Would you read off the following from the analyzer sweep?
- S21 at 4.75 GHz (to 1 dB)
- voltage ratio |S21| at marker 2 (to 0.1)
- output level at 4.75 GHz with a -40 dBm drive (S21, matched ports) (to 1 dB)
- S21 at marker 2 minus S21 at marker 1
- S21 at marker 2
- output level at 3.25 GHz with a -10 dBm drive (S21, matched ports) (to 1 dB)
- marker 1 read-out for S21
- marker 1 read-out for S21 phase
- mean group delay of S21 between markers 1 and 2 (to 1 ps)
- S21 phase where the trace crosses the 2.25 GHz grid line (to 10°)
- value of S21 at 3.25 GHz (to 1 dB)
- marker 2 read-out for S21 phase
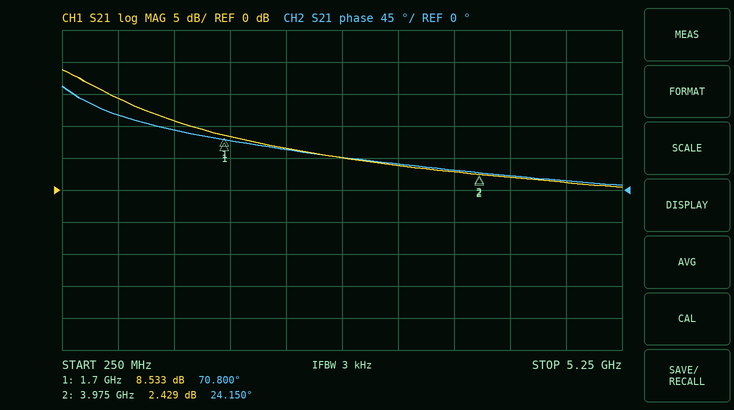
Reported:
1 dB
1.3
-39 dBm
-6.104 dB
2.429 dB
-6 dBm
8.533 dB
70.800°
57 ps
60°
4 dB
24.150°
